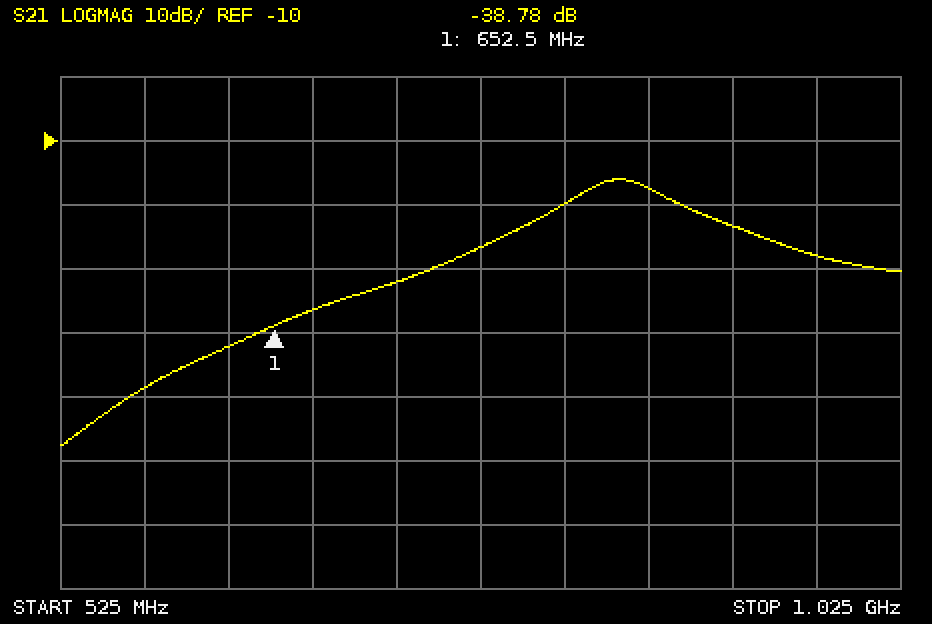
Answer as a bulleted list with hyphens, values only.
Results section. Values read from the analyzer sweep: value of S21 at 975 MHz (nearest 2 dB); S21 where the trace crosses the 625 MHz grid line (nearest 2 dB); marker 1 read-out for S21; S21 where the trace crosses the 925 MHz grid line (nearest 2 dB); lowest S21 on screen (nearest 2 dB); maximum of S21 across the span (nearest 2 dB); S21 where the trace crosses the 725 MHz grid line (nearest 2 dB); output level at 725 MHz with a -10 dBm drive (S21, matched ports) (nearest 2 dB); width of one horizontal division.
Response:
- -28 dB
- -42 dB
- -38.78 dB
- -24 dB
- -58 dB
- -16 dB
- -32 dB
- -42 dBm
- 50 MHz
